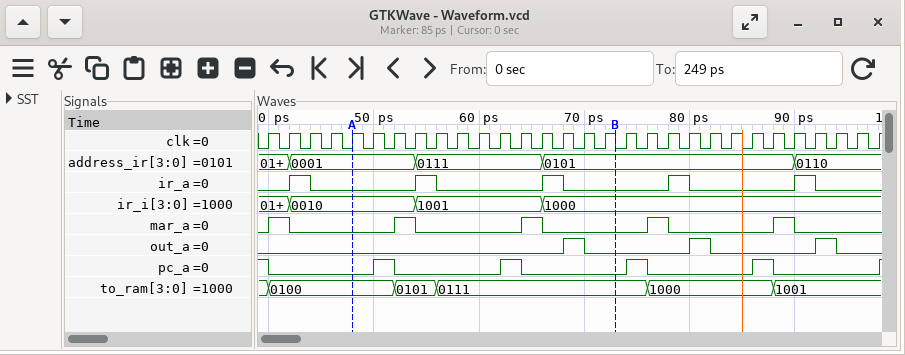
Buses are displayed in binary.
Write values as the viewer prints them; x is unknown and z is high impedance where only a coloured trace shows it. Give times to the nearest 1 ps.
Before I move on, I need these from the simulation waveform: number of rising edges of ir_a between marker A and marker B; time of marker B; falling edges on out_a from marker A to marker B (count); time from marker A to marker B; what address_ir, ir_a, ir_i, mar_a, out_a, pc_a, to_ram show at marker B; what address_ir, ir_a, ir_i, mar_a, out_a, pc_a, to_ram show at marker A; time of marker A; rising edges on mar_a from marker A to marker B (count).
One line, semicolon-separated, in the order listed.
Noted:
2; 73 ps; 1; 25 ps; address_ir=0101, ir_a=0, ir_i=1000, mar_a=0, out_a=0, pc_a=0, to_ram=0111; address_ir=0001, ir_a=0, ir_i=0010, mar_a=0, out_a=0, pc_a=0, to_ram=0100; 48 ps; 2
